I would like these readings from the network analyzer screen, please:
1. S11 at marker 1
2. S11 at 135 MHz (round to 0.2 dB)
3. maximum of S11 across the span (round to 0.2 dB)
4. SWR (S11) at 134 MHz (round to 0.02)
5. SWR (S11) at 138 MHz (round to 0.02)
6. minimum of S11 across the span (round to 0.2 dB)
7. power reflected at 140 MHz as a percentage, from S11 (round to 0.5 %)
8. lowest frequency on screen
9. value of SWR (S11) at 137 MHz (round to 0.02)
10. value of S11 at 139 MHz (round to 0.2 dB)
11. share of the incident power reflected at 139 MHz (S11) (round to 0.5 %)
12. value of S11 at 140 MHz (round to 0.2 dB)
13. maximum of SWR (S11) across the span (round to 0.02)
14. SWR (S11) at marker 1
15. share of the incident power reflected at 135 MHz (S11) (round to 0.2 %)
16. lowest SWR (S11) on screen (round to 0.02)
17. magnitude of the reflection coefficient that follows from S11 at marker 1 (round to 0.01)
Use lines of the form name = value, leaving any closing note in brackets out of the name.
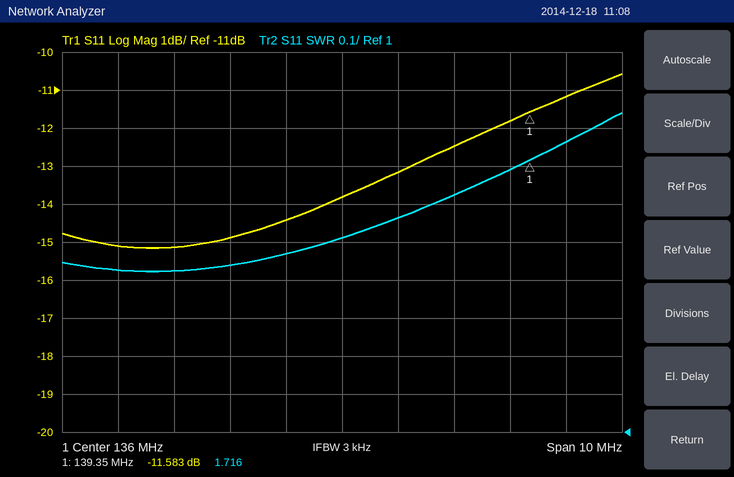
S11 at marker 1 = -11.583 dB
S11 at 135 MHz = -14.4 dB
maximum of S11 across the span = -10.6 dB
SWR (S11) at 134 MHz = 1.44
SWR (S11) at 138 MHz = 1.62
minimum of S11 across the span = -15.2 dB
power reflected at 140 MHz as a percentage, from S11 = 7.5 %
lowest frequency on screen = 131 MHz
value of SWR (S11) at 137 MHz = 1.56
value of S11 at 139 MHz = -11.8 dB
share of the incident power reflected at 139 MHz (S11) = 6.5 %
value of S11 at 140 MHz = -11.2 dB
maximum of SWR (S11) across the span = 1.84
SWR (S11) at marker 1 = 1.716
share of the incident power reflected at 135 MHz (S11) = 3.6 %
lowest SWR (S11) on screen = 1.42
magnitude of the reflection coefficient that follows from S11 at marker 1 = 0.26
